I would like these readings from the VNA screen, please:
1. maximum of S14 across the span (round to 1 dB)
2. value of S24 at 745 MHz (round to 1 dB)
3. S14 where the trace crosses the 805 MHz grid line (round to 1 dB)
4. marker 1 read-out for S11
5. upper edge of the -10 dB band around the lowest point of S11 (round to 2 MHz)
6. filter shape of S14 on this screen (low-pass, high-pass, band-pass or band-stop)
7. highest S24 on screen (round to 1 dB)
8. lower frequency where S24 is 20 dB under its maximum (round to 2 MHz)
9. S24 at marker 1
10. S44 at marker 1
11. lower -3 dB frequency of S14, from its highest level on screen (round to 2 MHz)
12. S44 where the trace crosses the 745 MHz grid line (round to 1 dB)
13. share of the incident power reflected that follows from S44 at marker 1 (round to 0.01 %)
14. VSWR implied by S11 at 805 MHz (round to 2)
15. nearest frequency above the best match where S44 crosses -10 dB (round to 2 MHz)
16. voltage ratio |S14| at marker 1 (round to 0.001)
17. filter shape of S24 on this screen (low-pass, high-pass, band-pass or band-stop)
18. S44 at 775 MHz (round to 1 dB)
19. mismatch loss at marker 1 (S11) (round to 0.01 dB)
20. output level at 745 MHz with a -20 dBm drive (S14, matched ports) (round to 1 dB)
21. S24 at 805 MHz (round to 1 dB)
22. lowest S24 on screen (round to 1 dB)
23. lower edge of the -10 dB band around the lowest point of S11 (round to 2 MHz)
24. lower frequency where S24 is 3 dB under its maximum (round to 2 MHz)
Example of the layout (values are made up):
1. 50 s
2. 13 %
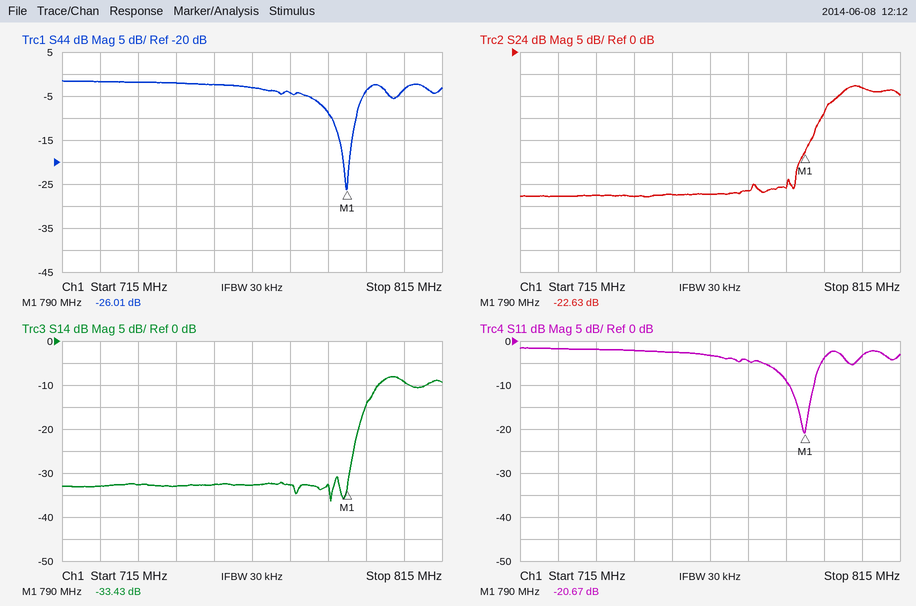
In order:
1. -8 dB
2. -33 dB
3. -9 dB
4. -20.67 dB
5. 792 MHz
6. high-pass
7. -8 dB
8. 788 MHz
9. -22.63 dB
10. -26.01 dB
11. 798 MHz
12. -2 dB
13. 0.25 %
14. 6
15. 792 MHz
16. 0.021
17. high-pass
18. -4 dB
19. 0.04 dB
20. -53 dBm
21. -8 dB
22. -33 dB
23. 786 MHz
24. 798 MHz
